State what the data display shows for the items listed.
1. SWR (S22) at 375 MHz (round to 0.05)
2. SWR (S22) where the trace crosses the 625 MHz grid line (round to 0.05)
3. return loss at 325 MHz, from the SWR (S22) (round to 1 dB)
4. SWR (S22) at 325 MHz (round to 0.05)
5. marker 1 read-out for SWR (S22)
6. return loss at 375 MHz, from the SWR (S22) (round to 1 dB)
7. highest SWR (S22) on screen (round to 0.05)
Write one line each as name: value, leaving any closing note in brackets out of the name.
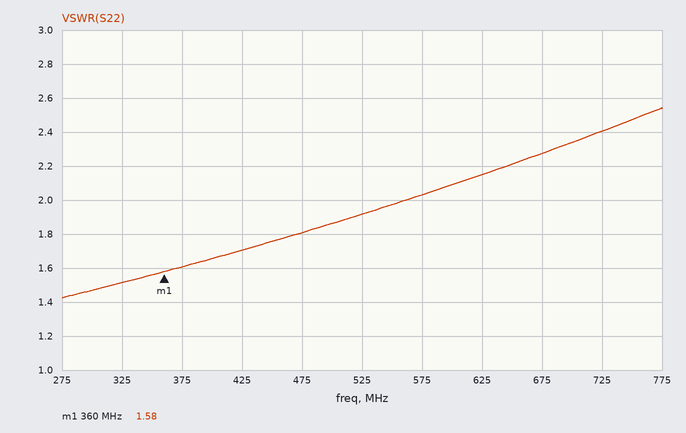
SWR (S22) at 375 MHz: 1.60
SWR (S22) where the trace crosses the 625 MHz grid line: 2.15
return loss at 325 MHz, from the SWR (S22): 14 dB
SWR (S22) at 325 MHz: 1.50
marker 1 read-out for SWR: 1.58
return loss at 375 MHz, from the SWR (S22): 13 dB
highest SWR (S22) on screen: 2.55
